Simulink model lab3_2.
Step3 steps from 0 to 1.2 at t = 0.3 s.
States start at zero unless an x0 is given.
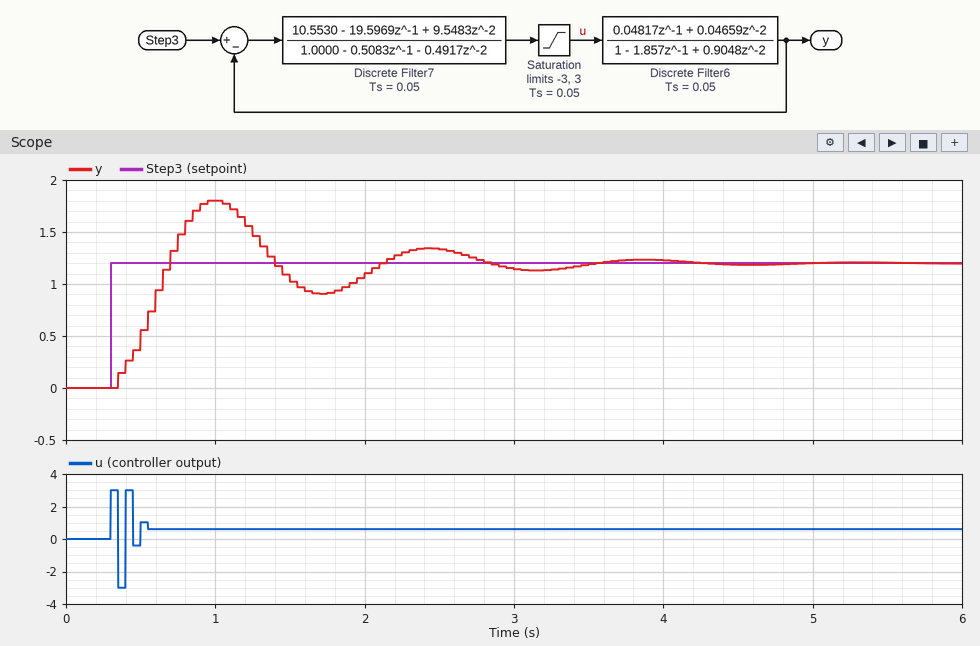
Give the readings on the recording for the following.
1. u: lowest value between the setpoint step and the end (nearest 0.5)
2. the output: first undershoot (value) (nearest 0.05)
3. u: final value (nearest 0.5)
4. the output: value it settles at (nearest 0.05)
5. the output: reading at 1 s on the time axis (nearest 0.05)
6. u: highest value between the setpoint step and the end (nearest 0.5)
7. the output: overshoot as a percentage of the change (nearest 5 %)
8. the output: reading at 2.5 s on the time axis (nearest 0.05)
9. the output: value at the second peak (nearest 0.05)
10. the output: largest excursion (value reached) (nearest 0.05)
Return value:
-3.0
0.90
0.5
1.20
1.80
3.0
50 %
1.35
1.35
1.80
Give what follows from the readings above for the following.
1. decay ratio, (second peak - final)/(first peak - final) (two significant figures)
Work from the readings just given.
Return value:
0.25
